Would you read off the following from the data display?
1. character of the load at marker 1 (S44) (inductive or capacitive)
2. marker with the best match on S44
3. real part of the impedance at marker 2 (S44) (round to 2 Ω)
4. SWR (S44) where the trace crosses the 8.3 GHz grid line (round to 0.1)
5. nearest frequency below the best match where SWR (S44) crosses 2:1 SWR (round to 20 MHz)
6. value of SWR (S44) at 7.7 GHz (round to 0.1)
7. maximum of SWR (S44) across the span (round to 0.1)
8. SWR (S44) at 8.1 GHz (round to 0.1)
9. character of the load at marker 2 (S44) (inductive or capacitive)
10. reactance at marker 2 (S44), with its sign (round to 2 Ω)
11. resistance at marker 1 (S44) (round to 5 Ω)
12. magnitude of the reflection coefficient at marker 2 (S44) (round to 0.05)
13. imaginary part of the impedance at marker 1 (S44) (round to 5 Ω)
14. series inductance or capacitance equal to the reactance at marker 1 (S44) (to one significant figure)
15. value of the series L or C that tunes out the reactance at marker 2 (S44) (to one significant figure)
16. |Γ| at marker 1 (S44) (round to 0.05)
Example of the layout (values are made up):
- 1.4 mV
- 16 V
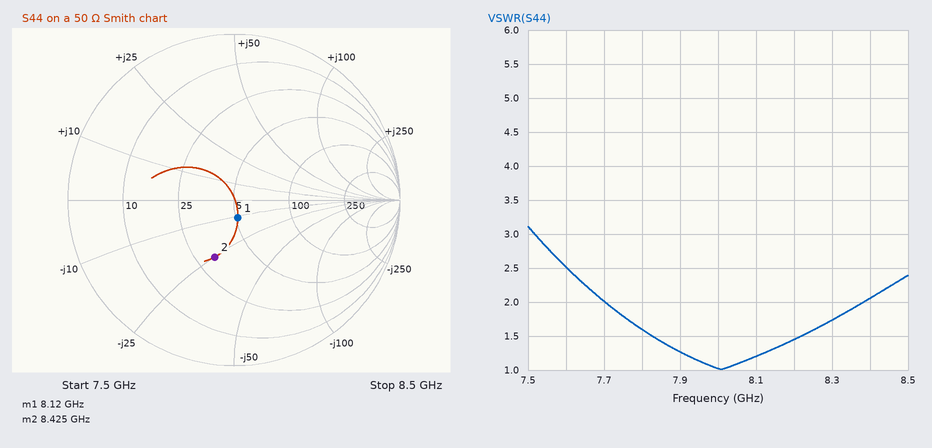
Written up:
- capacitive
- marker 1
- 32 Ω
- 1.7
- 7.70 GHz
- 2.0
- 3.1
- 1.2
- capacitive
- -26 Ω
- 50 Ω
- 0.35
- -10 Ω
- 2 pF
- 500 pH
- 0.10
